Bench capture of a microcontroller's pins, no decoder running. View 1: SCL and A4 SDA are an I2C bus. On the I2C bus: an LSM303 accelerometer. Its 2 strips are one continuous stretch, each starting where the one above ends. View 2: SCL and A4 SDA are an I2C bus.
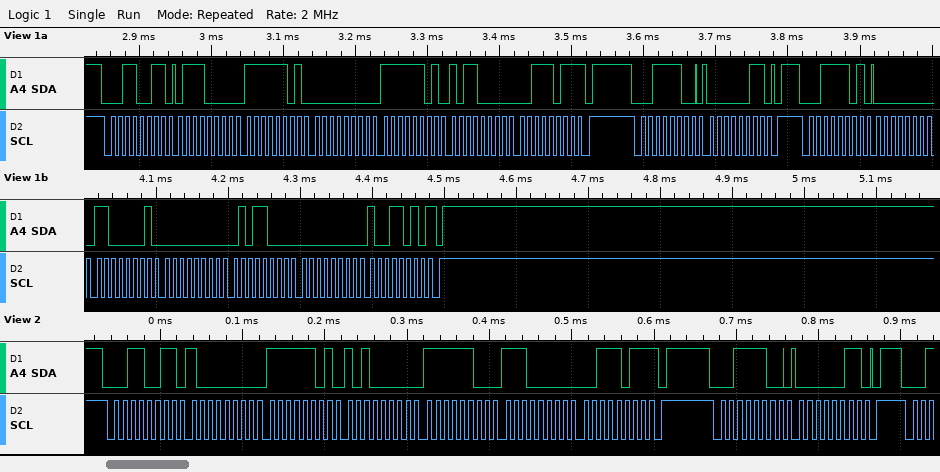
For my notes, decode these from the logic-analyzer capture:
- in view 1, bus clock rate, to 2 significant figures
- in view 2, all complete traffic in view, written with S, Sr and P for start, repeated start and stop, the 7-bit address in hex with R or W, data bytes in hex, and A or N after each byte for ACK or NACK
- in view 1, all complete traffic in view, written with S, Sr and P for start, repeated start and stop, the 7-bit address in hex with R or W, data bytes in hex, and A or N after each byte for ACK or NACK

100 kHz
S 19R A 80 A FD A A0 A FC A E0 A 3B N P S 1EW A 03 A P
S 19R A 70 A FD A 00 A FD A B0 A 3B N P S 1EW A 03 A P S 1ER A 00 A C1 A 00 A 58 A 00 A 9A N P
